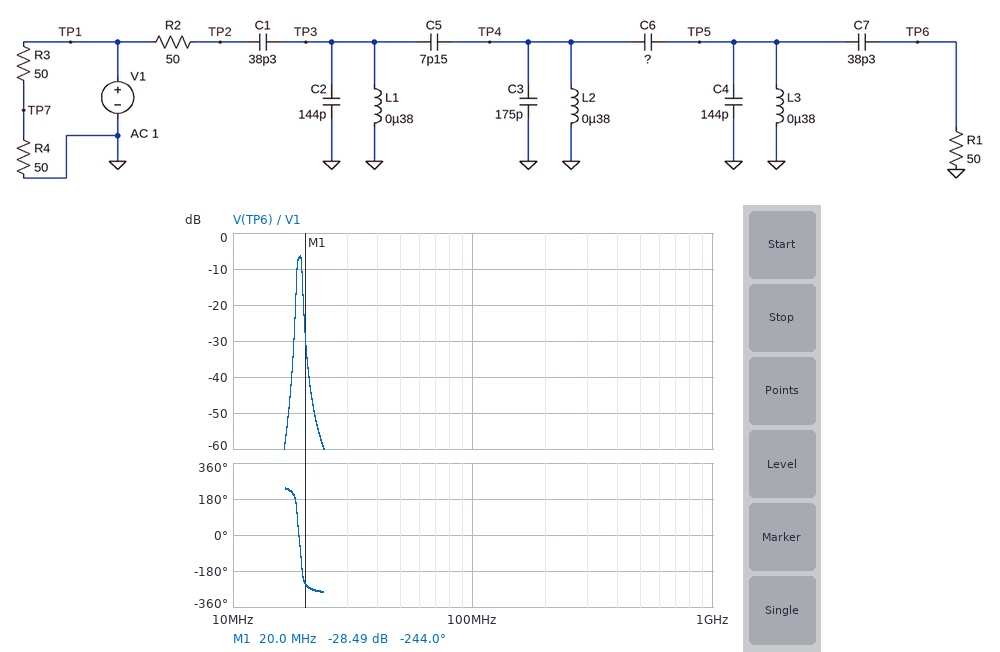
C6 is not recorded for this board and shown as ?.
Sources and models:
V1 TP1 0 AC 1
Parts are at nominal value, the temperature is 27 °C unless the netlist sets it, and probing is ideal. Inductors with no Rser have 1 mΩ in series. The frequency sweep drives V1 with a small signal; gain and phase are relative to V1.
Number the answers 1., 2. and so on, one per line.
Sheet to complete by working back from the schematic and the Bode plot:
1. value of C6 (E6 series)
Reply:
1. 4.7 pF
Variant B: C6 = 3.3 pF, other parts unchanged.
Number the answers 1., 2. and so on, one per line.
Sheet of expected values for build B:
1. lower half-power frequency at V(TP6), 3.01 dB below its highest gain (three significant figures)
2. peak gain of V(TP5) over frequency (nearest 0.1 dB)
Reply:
1. 18.7 MHz
2. 5.4 dB
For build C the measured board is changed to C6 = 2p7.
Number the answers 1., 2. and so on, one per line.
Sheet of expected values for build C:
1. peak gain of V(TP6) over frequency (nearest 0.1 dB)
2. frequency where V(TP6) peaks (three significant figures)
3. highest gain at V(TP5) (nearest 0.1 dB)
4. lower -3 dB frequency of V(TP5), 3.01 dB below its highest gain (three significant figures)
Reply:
1. -8.5 dB
2. 19.2 MHz
3. 4.5 dB
4. 18.8 MHz
